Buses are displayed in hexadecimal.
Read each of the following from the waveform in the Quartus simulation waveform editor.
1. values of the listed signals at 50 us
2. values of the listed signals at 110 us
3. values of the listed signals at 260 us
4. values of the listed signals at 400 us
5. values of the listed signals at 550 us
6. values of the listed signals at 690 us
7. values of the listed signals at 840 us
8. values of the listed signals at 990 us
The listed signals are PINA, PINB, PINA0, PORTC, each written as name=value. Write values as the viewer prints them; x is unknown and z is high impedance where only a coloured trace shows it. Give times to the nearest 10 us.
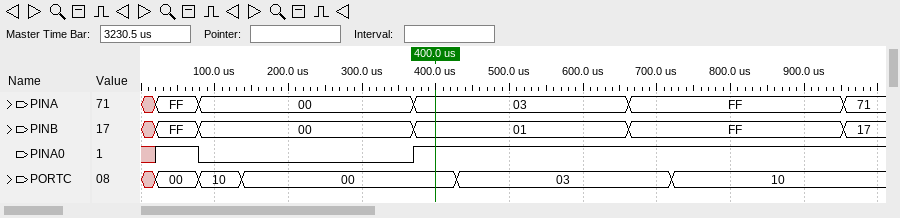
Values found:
PINA=FF, PINB=FF, PINA0=1, PORTC=00
PINA=00, PINB=00, PINA0=0, PORTC=10
PINA=00, PINB=00, PINA0=0, PORTC=00
PINA=03, PINB=01, PINA0=1, PORTC=00
PINA=03, PINB=01, PINA0=1, PORTC=03
PINA=FF, PINB=FF, PINA0=1, PORTC=03
PINA=FF, PINB=FF, PINA0=1, PORTC=10
PINA=71, PINB=17, PINA0=1, PORTC=10
